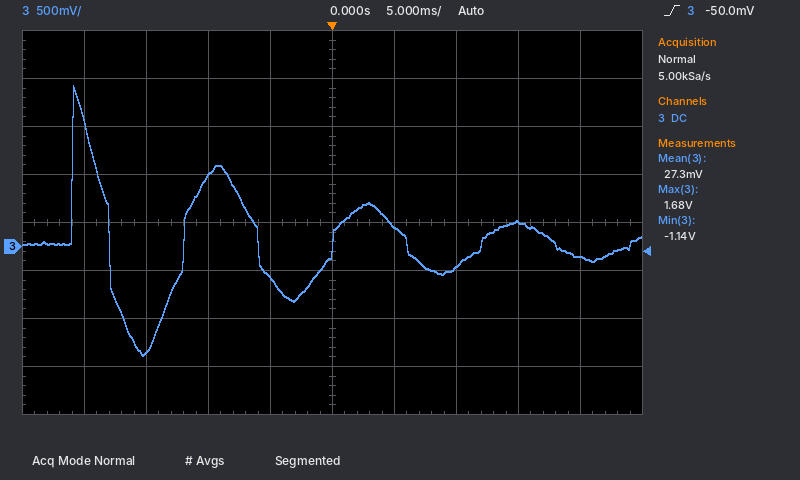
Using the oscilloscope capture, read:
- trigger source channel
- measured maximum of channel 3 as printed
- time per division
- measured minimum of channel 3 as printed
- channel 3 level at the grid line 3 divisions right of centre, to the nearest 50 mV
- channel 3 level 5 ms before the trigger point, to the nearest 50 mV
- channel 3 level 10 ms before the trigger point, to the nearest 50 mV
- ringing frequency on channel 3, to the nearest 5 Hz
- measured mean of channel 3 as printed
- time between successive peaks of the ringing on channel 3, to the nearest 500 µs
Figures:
channel 3
1.68 V
5 ms
-1.14 V
250 mV
-300 mV
750 mV
85 Hz
27.3 mV
12.0 ms
